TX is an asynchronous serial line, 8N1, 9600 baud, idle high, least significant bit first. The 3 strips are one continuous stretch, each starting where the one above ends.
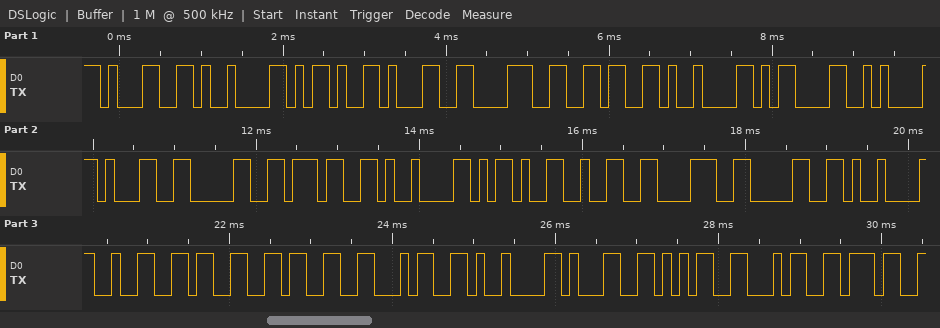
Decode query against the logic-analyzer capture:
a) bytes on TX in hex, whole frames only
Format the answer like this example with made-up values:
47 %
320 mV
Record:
31 09 2D 31 38 36 09 0D 0A 31 30 37 09 2D 32 38 30 09 32 33 33 34 09 31 35 34 37
